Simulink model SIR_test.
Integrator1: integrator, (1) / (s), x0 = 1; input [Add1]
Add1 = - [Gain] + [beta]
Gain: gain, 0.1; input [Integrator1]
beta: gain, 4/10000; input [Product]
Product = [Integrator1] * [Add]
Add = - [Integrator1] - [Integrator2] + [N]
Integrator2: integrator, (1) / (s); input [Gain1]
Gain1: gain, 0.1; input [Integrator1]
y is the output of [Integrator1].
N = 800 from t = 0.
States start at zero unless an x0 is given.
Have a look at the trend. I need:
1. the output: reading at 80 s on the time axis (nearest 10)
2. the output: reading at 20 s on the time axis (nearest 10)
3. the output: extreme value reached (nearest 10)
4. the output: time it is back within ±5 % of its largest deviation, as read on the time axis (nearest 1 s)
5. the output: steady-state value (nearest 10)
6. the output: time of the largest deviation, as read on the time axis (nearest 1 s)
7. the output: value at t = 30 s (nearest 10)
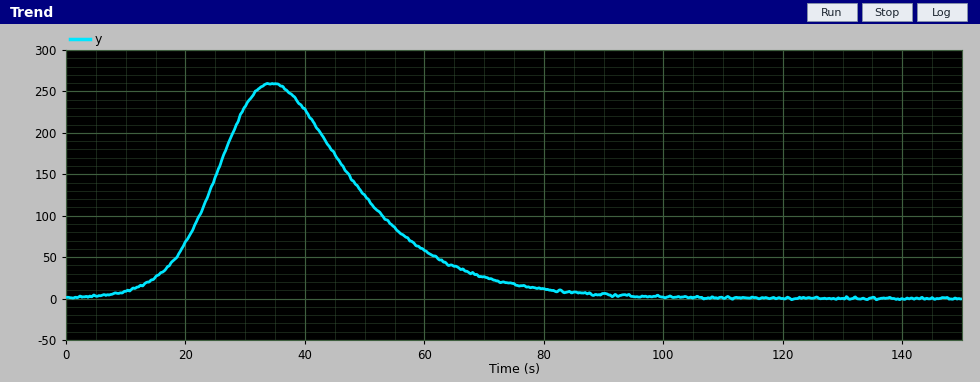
10
70
260
78 s
0
34 s
230
